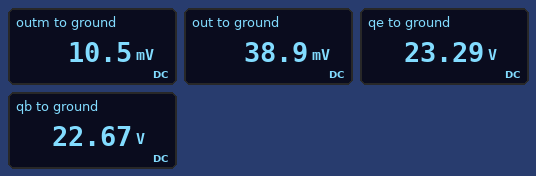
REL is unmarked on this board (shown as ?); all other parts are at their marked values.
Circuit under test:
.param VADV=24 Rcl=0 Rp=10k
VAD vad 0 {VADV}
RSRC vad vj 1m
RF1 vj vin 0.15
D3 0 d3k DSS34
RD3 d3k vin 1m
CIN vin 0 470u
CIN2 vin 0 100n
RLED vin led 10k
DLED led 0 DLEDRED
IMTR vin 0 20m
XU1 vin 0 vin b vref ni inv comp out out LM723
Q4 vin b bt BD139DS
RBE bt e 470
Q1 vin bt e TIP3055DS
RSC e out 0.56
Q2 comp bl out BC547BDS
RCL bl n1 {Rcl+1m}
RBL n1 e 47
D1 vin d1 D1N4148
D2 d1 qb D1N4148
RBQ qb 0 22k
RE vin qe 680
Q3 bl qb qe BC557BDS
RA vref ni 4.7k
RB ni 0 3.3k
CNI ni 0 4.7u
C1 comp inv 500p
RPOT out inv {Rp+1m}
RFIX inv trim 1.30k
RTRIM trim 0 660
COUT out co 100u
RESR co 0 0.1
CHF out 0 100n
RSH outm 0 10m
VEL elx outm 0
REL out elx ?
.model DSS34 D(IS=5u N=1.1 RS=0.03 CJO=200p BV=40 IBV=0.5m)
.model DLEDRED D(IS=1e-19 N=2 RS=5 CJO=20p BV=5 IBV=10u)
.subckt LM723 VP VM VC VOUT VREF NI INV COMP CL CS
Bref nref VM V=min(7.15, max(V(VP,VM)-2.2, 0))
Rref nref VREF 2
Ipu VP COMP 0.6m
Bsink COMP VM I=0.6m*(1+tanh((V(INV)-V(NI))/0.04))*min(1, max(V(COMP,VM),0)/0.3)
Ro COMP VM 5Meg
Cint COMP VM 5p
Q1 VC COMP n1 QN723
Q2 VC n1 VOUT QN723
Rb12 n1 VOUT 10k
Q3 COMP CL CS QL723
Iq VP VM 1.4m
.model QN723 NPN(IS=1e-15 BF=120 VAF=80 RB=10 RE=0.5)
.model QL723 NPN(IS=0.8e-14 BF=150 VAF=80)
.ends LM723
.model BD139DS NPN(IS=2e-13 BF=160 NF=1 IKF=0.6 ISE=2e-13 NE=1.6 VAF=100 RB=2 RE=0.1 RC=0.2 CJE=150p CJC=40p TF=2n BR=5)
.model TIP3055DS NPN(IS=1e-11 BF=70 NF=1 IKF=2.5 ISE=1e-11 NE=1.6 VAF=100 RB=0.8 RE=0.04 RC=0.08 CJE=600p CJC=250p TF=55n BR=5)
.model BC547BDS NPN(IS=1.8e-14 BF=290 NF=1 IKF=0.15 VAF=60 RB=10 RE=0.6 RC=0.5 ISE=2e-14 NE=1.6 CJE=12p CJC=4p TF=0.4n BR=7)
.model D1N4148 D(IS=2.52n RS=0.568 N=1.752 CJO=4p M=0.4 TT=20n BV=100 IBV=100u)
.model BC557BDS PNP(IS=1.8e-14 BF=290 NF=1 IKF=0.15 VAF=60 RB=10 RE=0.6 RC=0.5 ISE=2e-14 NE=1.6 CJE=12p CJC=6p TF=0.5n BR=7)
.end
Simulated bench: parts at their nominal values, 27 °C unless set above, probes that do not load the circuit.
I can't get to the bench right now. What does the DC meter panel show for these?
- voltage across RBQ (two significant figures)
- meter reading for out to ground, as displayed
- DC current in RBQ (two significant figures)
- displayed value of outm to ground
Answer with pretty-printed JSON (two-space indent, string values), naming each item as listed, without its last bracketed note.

{
  "voltage across RBQ": "23 V",
  "meter reading for out to ground, as displayed": "38.9 mV",
  "DC current in RBQ": "1.0 mA",
  "displayed value of outm to ground": "10.5 mV"
}
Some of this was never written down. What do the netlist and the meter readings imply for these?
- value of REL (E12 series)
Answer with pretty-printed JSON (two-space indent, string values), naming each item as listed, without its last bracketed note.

{
  "value of REL": "0.027 Ω"
}
